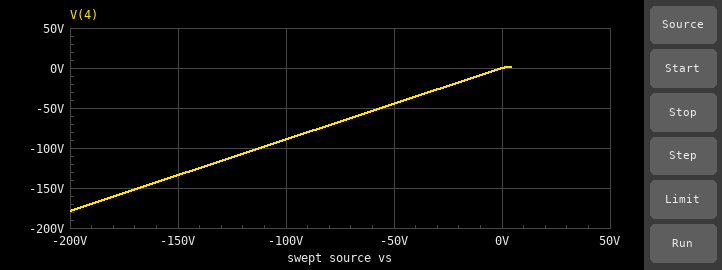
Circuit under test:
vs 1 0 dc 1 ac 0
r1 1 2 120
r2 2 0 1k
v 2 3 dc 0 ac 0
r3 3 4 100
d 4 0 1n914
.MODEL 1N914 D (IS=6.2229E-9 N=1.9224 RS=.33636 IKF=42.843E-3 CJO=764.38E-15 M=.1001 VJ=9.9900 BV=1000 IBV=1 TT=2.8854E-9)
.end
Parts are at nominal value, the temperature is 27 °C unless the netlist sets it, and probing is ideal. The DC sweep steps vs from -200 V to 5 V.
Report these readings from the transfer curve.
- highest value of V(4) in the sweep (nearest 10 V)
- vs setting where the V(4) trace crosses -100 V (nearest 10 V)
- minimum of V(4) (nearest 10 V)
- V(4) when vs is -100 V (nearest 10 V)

0 V
-110 V
-180 V
-90 V
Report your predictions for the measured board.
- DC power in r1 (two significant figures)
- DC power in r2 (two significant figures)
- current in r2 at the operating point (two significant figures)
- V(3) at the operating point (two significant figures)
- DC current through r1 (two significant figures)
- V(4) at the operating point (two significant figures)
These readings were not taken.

520 µW
560 µW
750 µA
750 mV
2.1 mA
620 mV
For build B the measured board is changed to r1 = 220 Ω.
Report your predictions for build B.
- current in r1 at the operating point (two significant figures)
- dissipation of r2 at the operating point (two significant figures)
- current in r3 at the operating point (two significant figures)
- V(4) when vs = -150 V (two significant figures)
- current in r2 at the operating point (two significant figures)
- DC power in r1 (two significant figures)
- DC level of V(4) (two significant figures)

1.5 mA
450 µW
810 µA
-120 V
670 µA
480 µW
590 mV
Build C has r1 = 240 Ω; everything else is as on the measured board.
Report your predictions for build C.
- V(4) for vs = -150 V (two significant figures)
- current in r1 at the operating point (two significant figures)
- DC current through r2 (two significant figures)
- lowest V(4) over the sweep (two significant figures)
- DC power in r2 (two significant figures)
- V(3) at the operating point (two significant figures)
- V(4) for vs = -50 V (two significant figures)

-120 V
1.4 mA
660 µA
-160 V
440 µW
660 mV
-40 V
